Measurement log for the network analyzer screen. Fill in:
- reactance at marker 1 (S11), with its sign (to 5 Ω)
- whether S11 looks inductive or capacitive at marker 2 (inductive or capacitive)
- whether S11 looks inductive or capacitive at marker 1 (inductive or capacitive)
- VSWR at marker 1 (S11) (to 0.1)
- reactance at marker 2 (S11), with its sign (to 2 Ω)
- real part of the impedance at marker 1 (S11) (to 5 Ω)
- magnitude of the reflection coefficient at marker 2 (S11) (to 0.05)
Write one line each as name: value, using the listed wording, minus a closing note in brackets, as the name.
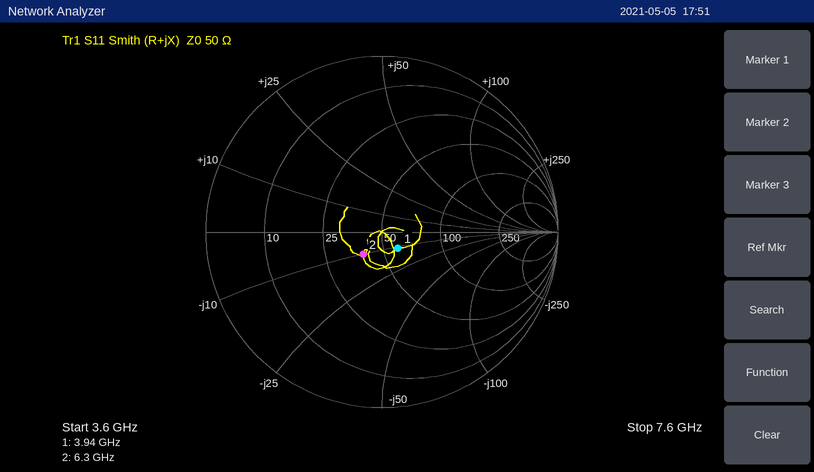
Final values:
reactance at marker 1 (S11), with its sign: -10 Ω
whether S11 looks inductive or capacitive at marker 2: capacitive
whether S11 looks inductive or capacitive at marker 1: capacitive
VSWR at marker 1 (S11): 1.3
reactance at marker 2 (S11), with its sign: -10 Ω
real part of the impedance at marker 1 (S11): 60 Ω
magnitude of the reflection coefficient at marker 2 (S11): 0.15
